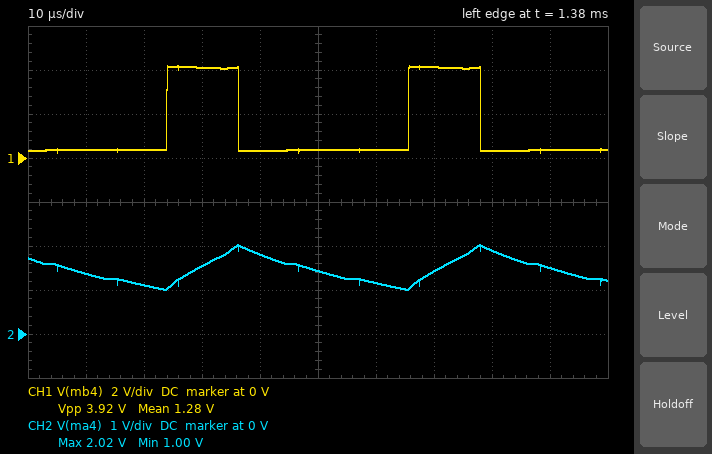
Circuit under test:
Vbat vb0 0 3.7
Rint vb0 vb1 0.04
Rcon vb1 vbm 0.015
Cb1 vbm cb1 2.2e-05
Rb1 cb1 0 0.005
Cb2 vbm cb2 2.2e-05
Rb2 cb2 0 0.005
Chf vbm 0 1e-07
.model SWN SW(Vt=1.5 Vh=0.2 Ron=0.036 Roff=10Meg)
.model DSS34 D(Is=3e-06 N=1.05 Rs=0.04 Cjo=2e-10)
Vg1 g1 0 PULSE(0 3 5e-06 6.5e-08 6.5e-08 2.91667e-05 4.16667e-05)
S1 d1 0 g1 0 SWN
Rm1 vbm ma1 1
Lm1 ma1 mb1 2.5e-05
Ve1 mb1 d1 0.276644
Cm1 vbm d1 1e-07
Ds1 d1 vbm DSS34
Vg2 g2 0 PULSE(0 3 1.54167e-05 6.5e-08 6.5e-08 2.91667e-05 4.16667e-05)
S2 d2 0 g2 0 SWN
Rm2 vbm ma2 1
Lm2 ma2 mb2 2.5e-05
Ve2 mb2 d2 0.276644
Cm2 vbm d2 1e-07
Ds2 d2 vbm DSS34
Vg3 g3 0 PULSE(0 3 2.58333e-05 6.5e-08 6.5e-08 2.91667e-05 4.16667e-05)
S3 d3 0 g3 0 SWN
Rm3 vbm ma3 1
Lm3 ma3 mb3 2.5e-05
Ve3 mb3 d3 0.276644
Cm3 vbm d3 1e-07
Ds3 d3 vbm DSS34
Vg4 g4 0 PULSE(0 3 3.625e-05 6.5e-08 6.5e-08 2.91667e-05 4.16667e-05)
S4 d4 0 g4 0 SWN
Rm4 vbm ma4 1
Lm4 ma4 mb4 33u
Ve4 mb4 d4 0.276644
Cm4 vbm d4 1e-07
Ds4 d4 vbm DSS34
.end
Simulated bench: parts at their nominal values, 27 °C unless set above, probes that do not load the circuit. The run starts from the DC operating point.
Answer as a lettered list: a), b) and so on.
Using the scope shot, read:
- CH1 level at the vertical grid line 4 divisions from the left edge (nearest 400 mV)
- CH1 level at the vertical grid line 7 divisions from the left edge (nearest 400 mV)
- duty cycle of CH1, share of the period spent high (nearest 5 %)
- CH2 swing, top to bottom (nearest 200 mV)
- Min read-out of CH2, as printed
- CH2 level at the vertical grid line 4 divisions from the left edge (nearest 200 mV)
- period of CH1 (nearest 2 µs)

a) 400 mV
b) 4.0 V
c) 30 %
d) 1.0 V
e) 1.00 V
f) 1.8 V
g) 42 µs
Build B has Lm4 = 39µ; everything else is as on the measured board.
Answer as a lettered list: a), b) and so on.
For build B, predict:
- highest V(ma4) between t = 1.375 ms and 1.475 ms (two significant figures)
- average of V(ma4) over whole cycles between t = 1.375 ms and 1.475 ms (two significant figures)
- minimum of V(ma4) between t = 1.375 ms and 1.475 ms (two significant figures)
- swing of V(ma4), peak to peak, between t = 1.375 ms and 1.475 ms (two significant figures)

a) 1.9 V
b) 1.5 V
c) 1.1 V
d) 880 mV
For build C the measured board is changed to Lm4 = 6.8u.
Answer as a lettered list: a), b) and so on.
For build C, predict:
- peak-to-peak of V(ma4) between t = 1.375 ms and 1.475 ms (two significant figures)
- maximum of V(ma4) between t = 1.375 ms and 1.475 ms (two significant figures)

a) 3.1 V
b) 3.5 V
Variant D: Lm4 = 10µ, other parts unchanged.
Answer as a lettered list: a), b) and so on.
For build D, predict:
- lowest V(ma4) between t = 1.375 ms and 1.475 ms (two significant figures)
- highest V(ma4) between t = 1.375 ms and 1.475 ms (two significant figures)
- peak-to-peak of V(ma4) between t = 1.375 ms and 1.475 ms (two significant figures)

a) 480 mV
b) 3.1 V
c) 2.6 V
